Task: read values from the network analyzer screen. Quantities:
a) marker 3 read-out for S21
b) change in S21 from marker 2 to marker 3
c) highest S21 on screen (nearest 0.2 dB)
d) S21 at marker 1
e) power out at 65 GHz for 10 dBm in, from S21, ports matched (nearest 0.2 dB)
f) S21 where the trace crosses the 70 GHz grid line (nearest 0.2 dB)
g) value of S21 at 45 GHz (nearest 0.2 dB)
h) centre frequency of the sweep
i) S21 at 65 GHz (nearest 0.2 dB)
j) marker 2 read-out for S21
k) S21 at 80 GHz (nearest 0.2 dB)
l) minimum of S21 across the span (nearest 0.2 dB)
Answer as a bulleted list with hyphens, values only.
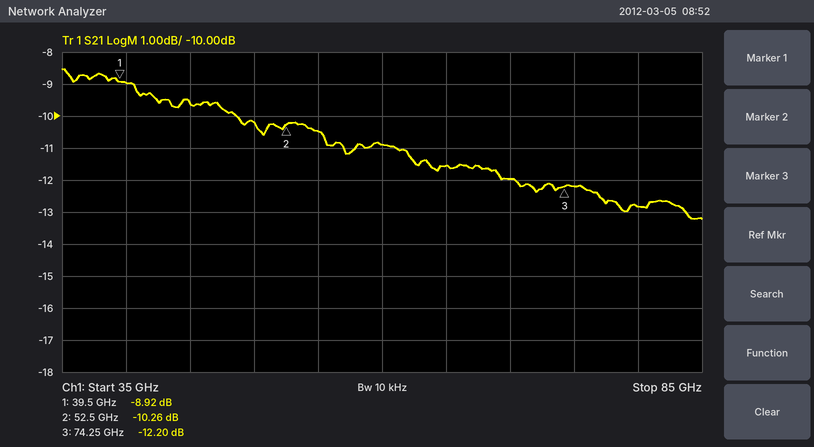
- -12.20 dB
- -1.94 dB
- -8.6 dB
- -8.92 dB
- -1.6 dBm
- -12.0 dB
- -9.6 dB
- 60 GHz
- -11.6 dB
- -10.26 dB
- -12.8 dB
- -13.2 dB
